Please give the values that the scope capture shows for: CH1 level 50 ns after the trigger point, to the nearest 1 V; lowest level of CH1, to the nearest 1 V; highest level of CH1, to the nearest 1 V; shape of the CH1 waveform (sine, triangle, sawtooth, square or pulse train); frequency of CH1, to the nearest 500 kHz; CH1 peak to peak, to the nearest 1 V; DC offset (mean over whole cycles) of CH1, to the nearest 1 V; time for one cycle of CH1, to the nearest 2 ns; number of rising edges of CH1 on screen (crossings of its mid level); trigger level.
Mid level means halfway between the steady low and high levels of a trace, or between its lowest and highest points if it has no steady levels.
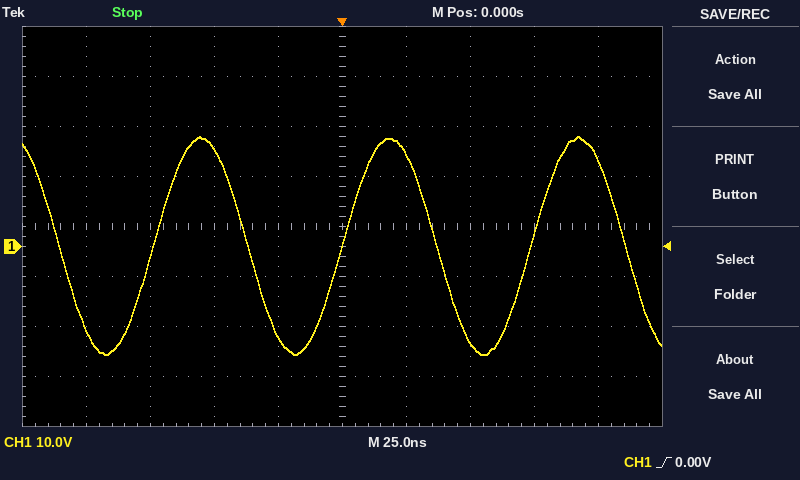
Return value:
-19 V
-22 V
22 V
sine
13.5 MHz
44 V
0 V
74 ns
3
0.00 V
